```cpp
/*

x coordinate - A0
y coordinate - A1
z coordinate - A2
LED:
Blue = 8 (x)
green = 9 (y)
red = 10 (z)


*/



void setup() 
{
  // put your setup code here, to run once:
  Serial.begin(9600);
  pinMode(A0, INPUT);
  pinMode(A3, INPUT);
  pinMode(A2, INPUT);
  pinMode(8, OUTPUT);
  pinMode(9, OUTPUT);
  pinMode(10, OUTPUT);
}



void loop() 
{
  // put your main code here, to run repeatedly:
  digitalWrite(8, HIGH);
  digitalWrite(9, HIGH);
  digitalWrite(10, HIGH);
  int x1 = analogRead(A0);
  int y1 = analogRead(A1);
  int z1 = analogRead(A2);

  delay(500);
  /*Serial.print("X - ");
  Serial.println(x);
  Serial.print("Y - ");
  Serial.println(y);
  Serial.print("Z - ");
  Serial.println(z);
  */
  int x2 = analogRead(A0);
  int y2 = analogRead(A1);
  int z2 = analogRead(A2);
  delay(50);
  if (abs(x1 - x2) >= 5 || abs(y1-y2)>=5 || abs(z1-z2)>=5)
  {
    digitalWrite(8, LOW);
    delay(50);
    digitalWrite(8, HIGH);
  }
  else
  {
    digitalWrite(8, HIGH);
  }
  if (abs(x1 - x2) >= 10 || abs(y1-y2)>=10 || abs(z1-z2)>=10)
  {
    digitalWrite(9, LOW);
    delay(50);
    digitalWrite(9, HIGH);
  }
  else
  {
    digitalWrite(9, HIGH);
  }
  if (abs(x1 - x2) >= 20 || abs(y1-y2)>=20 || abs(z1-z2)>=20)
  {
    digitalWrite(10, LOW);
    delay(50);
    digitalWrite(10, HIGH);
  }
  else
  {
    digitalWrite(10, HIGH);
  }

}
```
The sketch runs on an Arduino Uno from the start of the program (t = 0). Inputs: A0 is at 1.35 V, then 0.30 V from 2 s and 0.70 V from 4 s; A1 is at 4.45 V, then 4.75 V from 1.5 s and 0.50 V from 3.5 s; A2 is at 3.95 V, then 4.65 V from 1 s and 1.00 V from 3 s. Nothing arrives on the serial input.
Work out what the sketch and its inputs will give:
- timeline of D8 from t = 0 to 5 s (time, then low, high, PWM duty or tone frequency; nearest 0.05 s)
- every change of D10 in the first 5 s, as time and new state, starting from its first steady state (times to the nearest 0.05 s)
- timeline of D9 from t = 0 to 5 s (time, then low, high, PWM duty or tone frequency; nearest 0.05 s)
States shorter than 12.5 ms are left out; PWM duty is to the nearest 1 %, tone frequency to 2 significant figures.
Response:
0 s high; 1.1 s low; 1.15 s high; 1.8 s low; 1.85 s high; 2.5 s low; 2.55 s high; 3.2 s low; 3.25 s high; 3.9 s low; 3.95 s high
0 s high; 1.2 s low; 1.25 s high; 1.9 s low; 1.95 s high; 2.6 s low; 2.65 s high; 3.3 s low; 3.35 s high; 4 s low; 4.05 s high
0 s high; 1.15 s low; 1.2 s high; 1.85 s low; 1.9 s high; 2.55 s low; 2.6 s high; 3.25 s low; 3.3 s high; 3.95 s low; 4 s high
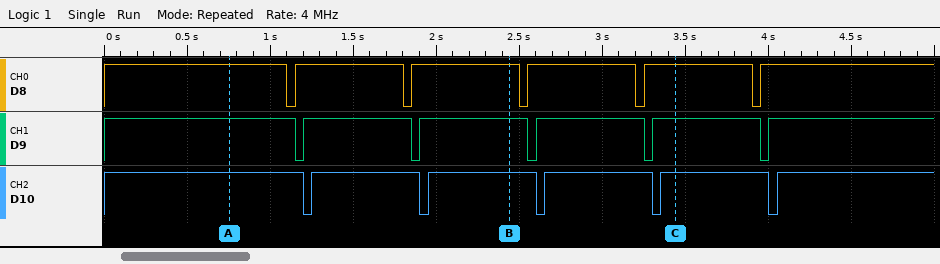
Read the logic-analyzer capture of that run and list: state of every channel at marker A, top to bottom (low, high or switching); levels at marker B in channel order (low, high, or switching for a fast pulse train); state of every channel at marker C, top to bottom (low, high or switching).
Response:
D8 high, D9 high, D10 high
D8 high, D9 high, D10 high
D8 high, D9 high, D10 high
